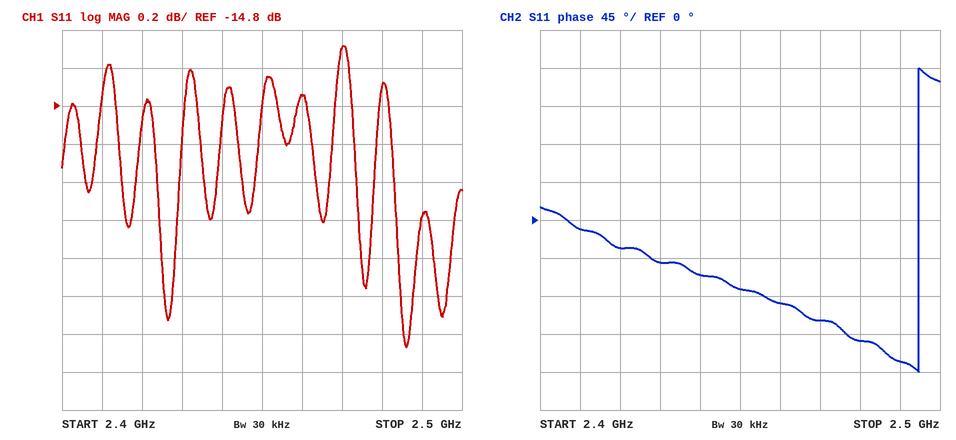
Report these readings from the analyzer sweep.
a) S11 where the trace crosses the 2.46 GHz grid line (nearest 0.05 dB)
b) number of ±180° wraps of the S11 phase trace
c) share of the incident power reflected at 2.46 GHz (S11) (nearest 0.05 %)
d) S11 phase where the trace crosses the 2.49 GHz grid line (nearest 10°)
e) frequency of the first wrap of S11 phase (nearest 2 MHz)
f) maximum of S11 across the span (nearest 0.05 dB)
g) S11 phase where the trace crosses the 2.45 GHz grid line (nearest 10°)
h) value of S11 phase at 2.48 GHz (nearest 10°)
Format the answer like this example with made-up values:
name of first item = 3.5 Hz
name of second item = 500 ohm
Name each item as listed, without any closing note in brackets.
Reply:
S11 where the trace crosses the 2.46 GHz grid line = -14.75 dB
number of ±180° wraps of the S11 phase trace = 1
share of the incident power reflected at 2.46 GHz (S11) = 3.35 %
S11 phase where the trace crosses the 2.49 GHz grid line = -170°
frequency of the first wrap of S11 phase = 2.494 GHz
maximum of S11 across the span = -14.50 dB
S11 phase where the trace crosses the 2.45 GHz grid line = -80°
value of S11 phase at 2.48 GHz = -140°
